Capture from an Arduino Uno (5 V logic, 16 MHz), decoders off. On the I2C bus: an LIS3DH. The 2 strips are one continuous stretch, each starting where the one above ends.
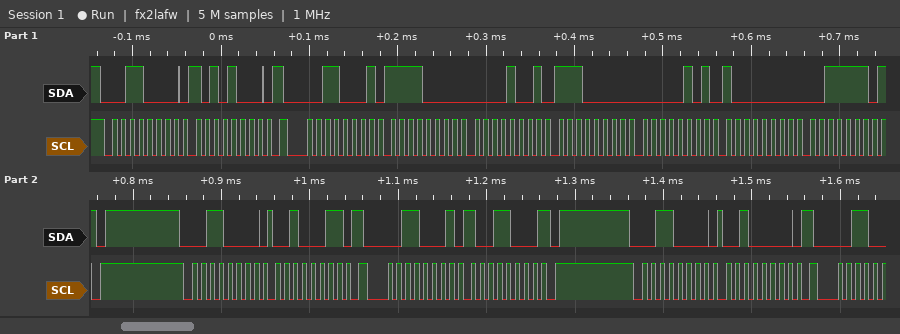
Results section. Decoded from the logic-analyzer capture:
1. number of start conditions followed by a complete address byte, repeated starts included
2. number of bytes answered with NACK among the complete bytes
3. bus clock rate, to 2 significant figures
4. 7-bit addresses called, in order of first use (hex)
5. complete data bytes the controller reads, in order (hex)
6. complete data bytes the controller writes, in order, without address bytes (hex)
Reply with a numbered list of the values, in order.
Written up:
1. 5
2. 2
3. 100 kHz
4. 0x18
5. F0 09 E0 05 80 3E 98
6. A8 23 20
